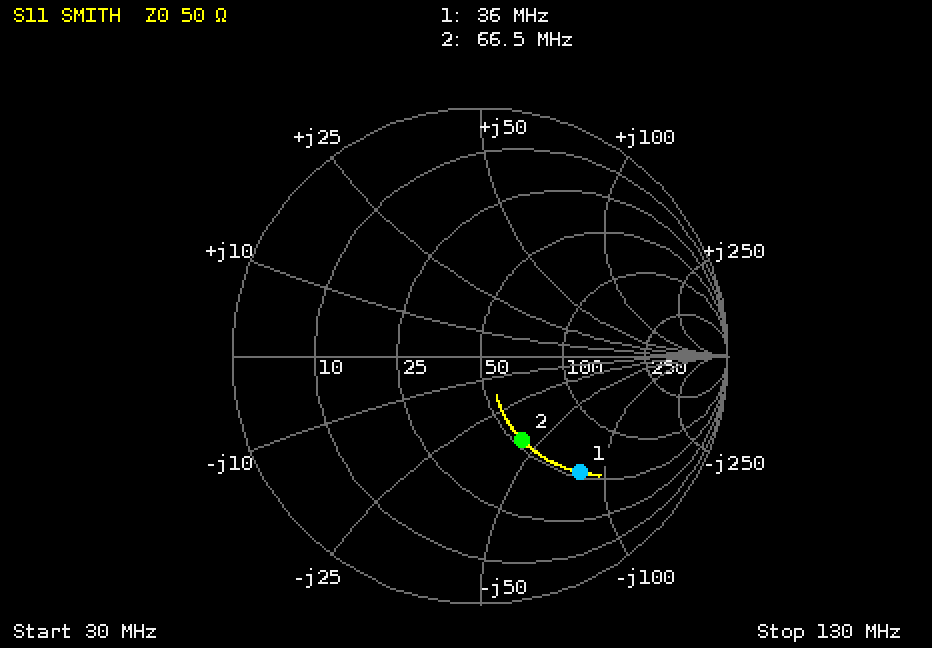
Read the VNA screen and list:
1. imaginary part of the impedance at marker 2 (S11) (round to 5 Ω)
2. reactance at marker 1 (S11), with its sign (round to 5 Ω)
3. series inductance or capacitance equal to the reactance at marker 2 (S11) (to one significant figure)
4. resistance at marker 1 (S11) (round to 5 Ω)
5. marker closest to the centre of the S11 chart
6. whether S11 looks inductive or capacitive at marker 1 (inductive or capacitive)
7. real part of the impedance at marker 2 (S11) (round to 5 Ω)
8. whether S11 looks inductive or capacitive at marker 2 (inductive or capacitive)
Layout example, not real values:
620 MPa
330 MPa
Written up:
-40 Ω
-80 Ω
60 pF
55 Ω
marker 2
capacitive
55 Ω
capacitive
